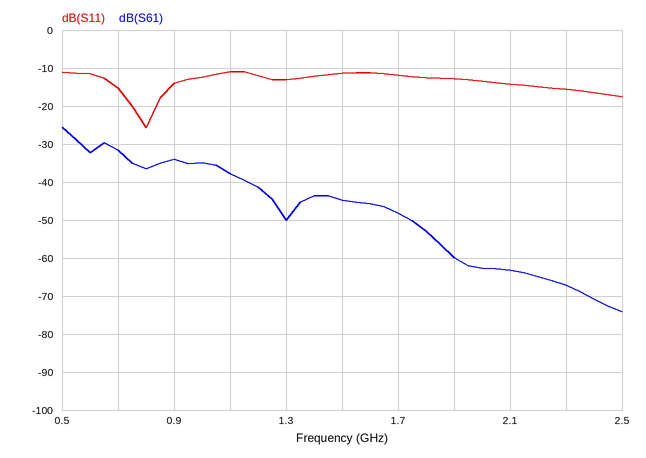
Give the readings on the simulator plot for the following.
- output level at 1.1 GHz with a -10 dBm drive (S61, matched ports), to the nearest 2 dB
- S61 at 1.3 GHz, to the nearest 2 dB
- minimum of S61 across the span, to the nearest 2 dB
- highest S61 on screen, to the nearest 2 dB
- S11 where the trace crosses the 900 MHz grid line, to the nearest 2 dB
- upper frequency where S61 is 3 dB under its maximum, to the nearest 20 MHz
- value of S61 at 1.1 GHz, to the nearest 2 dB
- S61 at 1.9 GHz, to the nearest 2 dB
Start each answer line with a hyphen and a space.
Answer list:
- -48 dBm
- -50 dB
- -74 dB
- -26 dB
- -14 dB
- 540 MHz
- -38 dB
- -60 dB
